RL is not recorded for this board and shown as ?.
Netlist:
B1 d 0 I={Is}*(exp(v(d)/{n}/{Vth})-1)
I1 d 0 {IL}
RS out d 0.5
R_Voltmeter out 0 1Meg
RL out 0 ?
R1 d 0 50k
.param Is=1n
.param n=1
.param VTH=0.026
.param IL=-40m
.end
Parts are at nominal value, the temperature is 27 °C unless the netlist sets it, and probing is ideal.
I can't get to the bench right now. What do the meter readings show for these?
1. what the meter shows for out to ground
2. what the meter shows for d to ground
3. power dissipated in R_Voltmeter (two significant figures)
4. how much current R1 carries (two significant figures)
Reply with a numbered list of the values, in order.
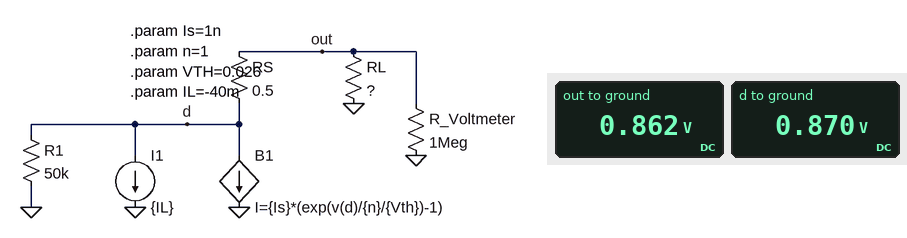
1. 0.862 V
2. 0.870 V
3. 740 nW
4. 17 µA
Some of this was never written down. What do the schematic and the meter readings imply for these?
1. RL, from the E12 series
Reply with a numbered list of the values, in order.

1. 56 Ω
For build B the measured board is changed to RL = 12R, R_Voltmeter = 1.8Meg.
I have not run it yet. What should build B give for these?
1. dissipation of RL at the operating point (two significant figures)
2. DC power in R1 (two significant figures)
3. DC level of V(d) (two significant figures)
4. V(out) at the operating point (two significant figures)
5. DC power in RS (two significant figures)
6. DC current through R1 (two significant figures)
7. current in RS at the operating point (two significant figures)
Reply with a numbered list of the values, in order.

1. 15 mW
2. 3.9 µW
3. 440 mV
4. 420 mV
5. 620 µW
6. 8.8 µA
7. 35 mA
